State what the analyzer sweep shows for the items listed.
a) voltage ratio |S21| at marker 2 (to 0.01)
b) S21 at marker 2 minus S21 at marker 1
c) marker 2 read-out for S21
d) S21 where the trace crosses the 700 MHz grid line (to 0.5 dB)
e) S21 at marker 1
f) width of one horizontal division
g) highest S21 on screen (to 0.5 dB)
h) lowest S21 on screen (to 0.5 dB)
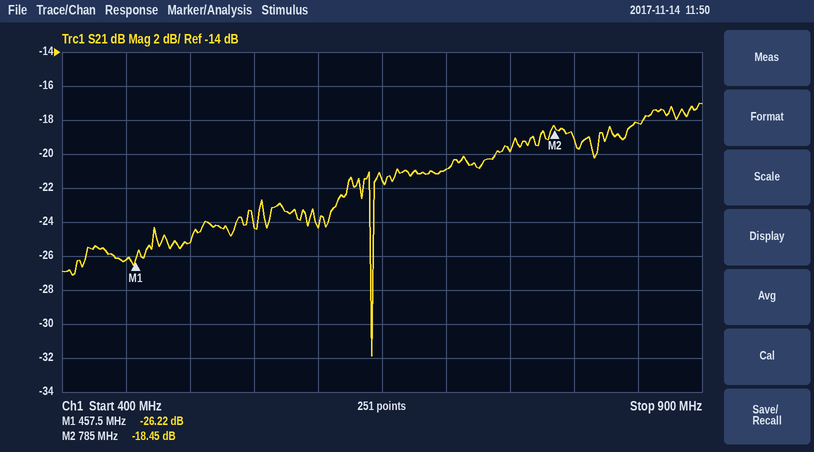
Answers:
0.12
7.77 dB
-18.45 dB
-21.0 dB
-26.22 dB
50 MHz
-17.0 dB
-32.0 dB
